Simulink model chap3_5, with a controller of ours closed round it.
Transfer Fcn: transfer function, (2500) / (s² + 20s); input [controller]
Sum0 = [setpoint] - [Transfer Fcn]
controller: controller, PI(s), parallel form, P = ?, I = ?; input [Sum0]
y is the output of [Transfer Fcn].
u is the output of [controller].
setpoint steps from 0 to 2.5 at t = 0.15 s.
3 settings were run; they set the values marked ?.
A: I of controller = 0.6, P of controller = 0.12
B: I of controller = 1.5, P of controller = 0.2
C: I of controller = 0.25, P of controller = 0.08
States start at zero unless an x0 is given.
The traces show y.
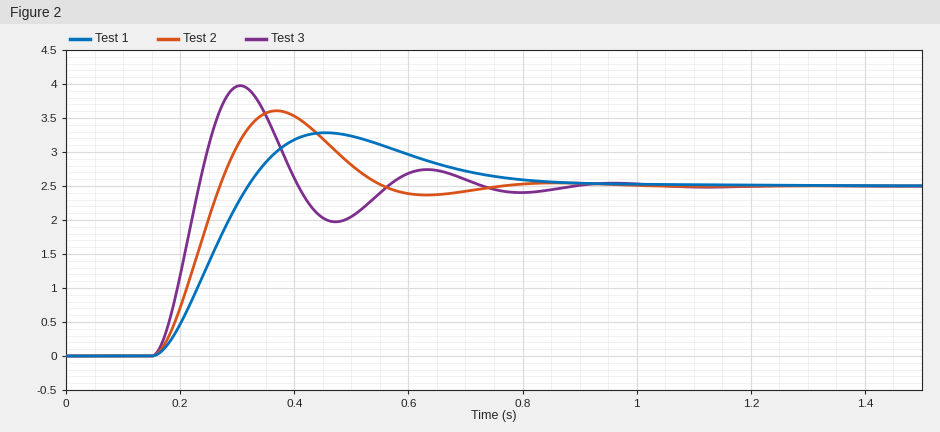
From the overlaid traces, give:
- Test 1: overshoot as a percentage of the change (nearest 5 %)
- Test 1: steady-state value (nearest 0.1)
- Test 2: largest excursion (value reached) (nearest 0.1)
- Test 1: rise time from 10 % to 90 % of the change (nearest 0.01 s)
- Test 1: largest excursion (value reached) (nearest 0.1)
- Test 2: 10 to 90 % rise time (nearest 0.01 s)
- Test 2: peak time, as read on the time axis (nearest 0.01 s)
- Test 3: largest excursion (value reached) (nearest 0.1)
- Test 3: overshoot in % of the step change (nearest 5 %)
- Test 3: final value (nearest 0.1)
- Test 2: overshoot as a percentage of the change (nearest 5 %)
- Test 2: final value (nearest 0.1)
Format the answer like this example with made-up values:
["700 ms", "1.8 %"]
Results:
["30 %", "2.5", "3.6", "0.12 s", "3.3", "0.08 s", "0.37 s", "4.0", "60 %", "2.5", "45 %", "2.5"]
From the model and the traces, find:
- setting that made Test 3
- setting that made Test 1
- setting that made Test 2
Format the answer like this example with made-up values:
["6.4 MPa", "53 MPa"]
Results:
["B", "C", "A"]
